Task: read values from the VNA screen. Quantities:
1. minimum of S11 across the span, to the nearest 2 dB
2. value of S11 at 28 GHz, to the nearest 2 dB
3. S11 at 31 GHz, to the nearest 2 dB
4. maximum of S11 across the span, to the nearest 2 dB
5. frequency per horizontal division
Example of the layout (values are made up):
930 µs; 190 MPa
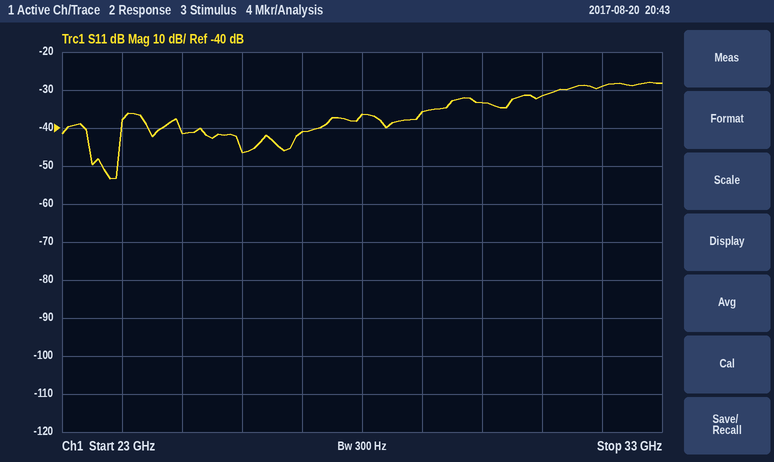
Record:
-54 dB; -36 dB; -32 dB; -28 dB; 1 GHz
